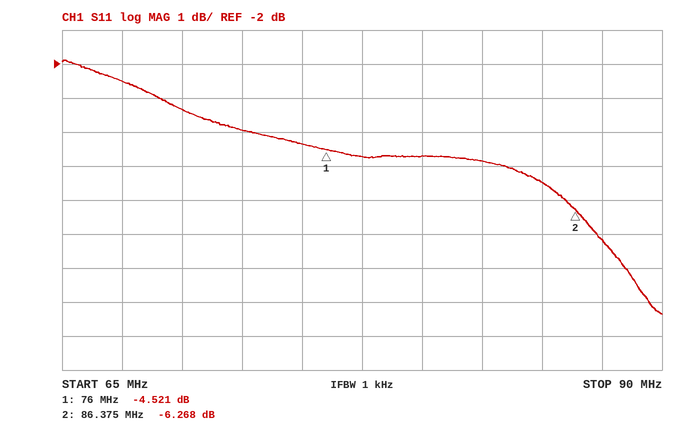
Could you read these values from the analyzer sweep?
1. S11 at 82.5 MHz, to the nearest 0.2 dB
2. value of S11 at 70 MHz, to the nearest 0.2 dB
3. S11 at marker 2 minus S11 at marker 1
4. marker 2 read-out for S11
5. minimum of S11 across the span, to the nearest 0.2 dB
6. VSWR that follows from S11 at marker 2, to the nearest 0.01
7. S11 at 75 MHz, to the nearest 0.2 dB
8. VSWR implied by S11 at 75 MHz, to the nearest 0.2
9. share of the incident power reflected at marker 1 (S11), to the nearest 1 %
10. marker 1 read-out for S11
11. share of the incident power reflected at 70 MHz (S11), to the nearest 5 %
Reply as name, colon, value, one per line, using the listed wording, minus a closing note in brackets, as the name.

S11 at 82.5 MHz, to the nearest 0.2 dB: -4.8 dB
value of S11 at 70 MHz, to the nearest 0.2 dB: -3.4 dB
S11 at marker 2 minus S11 at marker 1: -1.747 dB
marker 2 read-out for S11: -6.268 dB
minimum of S11 across the span, to the nearest 0.2 dB: -9.4 dB
VSWR that follows from S11 at marker 2, to the nearest 0.01: 2.89
S11 at 75 MHz, to the nearest 0.2 dB: -4.4 dB
VSWR implied by S11 at 75 MHz, to the nearest 0.2: 4.0
share of the incident power reflected at marker 1 (S11), to the nearest 1 %: 35 %
marker 1 read-out for S11: -4.521 dB
share of the incident power reflected at 70 MHz (S11), to the nearest 5 %: 45 %
